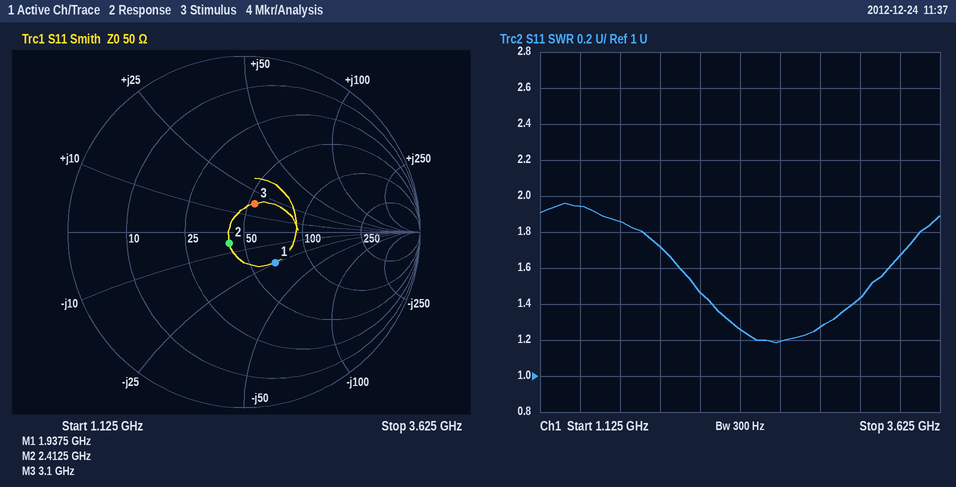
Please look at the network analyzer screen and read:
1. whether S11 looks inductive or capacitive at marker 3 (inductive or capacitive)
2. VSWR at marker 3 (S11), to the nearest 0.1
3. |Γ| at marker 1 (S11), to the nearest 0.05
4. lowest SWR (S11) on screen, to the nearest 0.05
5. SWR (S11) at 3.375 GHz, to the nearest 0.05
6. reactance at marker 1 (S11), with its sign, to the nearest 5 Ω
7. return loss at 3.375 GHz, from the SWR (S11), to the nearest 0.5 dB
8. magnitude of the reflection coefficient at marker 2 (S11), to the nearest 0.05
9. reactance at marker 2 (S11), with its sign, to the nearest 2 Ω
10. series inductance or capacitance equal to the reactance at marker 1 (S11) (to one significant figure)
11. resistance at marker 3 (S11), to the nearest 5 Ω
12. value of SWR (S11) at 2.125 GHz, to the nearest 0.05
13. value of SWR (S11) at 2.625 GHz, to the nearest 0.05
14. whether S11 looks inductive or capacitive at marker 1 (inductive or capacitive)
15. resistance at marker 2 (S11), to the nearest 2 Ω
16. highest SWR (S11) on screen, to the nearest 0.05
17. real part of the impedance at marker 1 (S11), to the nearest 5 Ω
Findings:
inductive
1.4
0.25
1.20
1.65
-25 Ω
12.0 dB
0.10
-6 Ω
3 pF
55 Ω
1.45
1.20
capacitive
42 Ω
1.95
65 Ω
